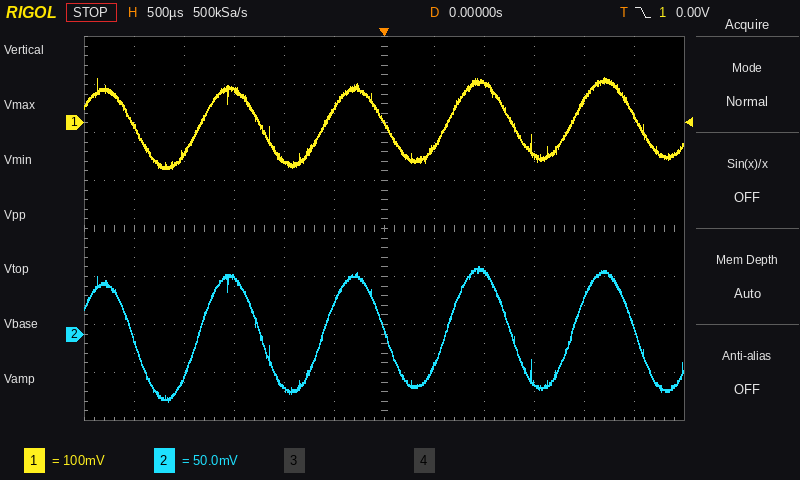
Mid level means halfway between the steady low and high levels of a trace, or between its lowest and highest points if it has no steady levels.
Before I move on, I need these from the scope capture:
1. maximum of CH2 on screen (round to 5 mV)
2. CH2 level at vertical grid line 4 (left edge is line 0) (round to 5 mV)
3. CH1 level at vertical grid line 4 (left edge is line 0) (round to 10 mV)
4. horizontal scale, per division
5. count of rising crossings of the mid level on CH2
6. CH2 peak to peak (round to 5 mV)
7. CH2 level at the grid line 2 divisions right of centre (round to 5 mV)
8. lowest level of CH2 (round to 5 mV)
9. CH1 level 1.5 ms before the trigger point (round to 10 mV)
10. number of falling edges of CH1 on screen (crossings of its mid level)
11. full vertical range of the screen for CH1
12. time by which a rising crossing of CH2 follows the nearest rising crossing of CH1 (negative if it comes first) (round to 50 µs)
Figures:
70 mV
-55 mV
-80 mV
500 µs
4
140 mV
65 mV
-70 mV
70 mV
5
800 mV
0 µs
